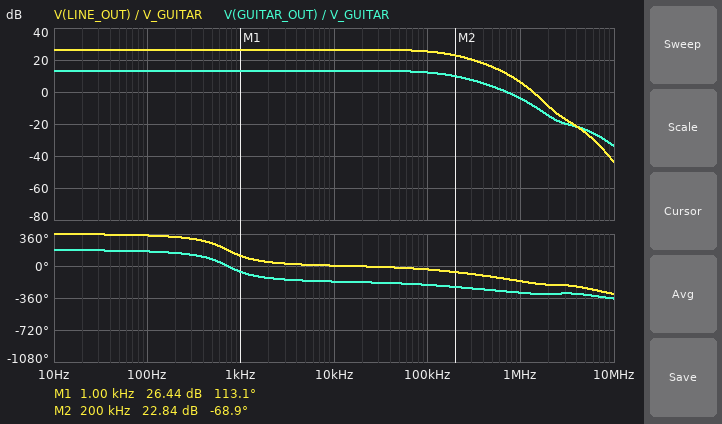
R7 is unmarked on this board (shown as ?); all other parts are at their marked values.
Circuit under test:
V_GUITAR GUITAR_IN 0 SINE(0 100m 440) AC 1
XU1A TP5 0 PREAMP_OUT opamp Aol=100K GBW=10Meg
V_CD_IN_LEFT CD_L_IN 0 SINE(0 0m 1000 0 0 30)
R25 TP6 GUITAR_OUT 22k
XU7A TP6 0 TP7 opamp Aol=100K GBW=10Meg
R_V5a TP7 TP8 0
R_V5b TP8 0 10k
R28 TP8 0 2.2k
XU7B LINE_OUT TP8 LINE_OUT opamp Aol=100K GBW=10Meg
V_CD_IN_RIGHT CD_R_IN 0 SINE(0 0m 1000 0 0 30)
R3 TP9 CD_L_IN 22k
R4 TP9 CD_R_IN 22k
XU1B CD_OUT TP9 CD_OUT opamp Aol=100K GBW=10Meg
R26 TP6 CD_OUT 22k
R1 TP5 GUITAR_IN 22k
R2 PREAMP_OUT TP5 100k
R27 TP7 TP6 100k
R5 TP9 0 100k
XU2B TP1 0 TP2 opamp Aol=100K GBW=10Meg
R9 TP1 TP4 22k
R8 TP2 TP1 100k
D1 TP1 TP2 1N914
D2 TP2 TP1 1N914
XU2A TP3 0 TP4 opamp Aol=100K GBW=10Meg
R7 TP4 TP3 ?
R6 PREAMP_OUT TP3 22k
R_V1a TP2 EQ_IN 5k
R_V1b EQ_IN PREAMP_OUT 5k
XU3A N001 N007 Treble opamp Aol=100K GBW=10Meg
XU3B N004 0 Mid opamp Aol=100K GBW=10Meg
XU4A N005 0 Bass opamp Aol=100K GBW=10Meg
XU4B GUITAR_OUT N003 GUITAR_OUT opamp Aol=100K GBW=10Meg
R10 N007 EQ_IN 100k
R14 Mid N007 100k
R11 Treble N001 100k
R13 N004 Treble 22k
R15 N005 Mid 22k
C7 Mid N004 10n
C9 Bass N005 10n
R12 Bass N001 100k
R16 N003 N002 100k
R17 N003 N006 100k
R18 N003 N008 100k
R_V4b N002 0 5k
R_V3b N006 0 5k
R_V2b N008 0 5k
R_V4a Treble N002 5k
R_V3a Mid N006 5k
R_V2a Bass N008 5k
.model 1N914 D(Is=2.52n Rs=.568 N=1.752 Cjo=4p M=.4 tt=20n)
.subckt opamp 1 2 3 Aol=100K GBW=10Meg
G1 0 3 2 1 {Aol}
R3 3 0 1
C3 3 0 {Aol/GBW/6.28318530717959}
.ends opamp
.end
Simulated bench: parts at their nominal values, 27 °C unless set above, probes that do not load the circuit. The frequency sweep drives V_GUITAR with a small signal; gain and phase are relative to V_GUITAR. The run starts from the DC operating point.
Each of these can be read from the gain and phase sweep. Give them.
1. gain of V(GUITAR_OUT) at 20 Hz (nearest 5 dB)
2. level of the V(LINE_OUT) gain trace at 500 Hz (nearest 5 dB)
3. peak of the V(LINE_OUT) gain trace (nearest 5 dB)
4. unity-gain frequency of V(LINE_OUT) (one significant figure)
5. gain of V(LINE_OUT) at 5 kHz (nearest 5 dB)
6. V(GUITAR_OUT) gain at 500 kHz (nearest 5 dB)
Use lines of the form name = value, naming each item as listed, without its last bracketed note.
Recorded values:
gain of V(GUITAR_OUT) at 20 Hz = 15 dB
level of the V(LINE_OUT) gain trace at 500 Hz = 25 dB
peak of the V(LINE_OUT) gain trace = 25 dB
unity-gain frequency of V(LINE_OUT) = 1 MHz
gain of V(LINE_OUT) at 5 kHz = 25 dB
V(GUITAR_OUT) gain at 500 kHz = 5 dB
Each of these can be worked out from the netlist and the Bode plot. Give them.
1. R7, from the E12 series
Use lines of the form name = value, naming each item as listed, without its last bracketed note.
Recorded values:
R7, from the E12 series = 56 kΩ
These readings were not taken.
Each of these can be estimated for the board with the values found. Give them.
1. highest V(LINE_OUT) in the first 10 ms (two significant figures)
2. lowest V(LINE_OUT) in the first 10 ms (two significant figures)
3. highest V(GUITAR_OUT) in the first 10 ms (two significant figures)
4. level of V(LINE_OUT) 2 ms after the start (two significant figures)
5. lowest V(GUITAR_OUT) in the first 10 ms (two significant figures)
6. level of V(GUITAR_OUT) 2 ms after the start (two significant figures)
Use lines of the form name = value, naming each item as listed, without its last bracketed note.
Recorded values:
highest V(LINE_OUT) in the first 10 ms = 380 mV
lowest V(LINE_OUT) in the first 10 ms = -380 mV
highest V(GUITAR_OUT) in the first 10 ms = 83 mV
level of V(LINE_OUT) 2 ms after the start = -310 mV
lowest V(GUITAR_OUT) in the first 10 ms = -83 mV
level of V(GUITAR_OUT) 2 ms after the start = 68 mV
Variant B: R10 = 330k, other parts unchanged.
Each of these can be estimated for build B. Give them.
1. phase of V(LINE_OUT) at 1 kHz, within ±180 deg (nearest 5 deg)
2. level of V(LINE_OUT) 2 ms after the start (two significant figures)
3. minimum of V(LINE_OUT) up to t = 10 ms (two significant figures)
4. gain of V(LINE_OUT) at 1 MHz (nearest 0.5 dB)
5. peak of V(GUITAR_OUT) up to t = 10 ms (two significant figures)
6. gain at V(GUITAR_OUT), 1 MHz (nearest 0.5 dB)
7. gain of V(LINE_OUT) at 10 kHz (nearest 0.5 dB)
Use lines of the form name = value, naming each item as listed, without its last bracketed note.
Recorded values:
phase of V(LINE_OUT) at 1 kHz, within ±180 deg = 125 deg
level of V(LINE_OUT) 2 ms after the start = -93 mV
minimum of V(LINE_OUT) up to t = 10 ms = -140 mV
gain of V(LINE_OUT) at 1 MHz = -0.5 dB
peak of V(GUITAR_OUT) up to t = 10 ms = 32 mV
gain at V(GUITAR_OUT), 1 MHz = -10.5 dB
gain of V(LINE_OUT) at 10 kHz = 20.0 dB
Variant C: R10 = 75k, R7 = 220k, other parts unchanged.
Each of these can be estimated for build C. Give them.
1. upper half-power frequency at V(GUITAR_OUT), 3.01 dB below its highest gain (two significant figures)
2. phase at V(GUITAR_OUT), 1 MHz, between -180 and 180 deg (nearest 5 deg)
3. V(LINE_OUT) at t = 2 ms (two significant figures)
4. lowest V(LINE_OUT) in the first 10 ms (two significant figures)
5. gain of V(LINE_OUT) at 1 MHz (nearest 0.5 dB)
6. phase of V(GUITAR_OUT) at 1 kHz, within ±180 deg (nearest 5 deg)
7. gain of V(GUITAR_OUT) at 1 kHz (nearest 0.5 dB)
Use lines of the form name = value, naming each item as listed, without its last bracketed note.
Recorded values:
upper half-power frequency at V(GUITAR_OUT), 3.01 dB below its highest gain = 130 kHz
phase at V(GUITAR_OUT), 1 MHz, between -180 and 180 deg = 10 deg
V(LINE_OUT) at t = 2 ms = -440 mV
lowest V(LINE_OUT) in the first 10 ms = -510 mV
gain of V(LINE_OUT) at 1 MHz = 15.0 dB
phase of V(GUITAR_OUT) at 1 kHz, within ±180 deg = -70 deg
gain of V(GUITAR_OUT) at 1 kHz = 26.5 dB
